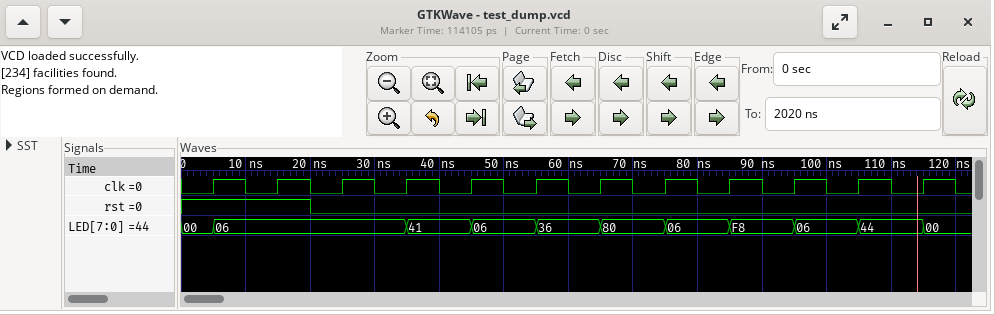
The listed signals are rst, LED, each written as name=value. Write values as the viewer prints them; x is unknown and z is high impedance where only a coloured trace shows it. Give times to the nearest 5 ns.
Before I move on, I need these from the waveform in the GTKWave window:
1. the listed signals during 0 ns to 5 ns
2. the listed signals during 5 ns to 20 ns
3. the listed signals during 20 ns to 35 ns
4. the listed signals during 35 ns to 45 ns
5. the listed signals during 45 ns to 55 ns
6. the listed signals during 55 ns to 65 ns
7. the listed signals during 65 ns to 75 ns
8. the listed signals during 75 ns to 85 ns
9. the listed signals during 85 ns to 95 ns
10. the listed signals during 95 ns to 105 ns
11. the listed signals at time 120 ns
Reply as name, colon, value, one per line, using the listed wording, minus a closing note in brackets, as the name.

the listed signals during 0 ns to 5 ns: rst=1, LED=00
the listed signals during 5 ns to 20 ns: rst=1, LED=06
the listed signals during 20 ns to 35 ns: rst=0, LED=06
the listed signals during 35 ns to 45 ns: rst=0, LED=41
the listed signals during 45 ns to 55 ns: rst=0, LED=06
the listed signals during 55 ns to 65 ns: rst=0, LED=36
the listed signals during 65 ns to 75 ns: rst=0, LED=80
the listed signals during 75 ns to 85 ns: rst=0, LED=06
the listed signals during 85 ns to 95 ns: rst=0, LED=F8
the listed signals during 95 ns to 105 ns: rst=0, LED=06
the listed signals at time 120 ns: rst=0, LED=00
